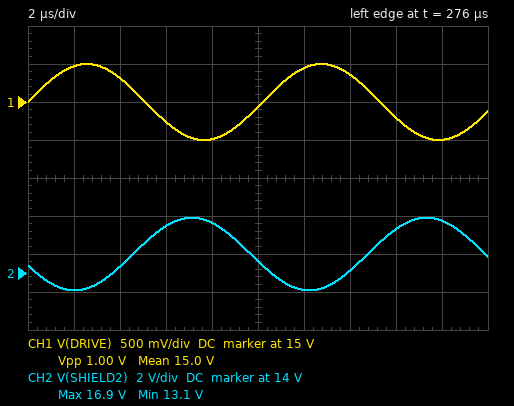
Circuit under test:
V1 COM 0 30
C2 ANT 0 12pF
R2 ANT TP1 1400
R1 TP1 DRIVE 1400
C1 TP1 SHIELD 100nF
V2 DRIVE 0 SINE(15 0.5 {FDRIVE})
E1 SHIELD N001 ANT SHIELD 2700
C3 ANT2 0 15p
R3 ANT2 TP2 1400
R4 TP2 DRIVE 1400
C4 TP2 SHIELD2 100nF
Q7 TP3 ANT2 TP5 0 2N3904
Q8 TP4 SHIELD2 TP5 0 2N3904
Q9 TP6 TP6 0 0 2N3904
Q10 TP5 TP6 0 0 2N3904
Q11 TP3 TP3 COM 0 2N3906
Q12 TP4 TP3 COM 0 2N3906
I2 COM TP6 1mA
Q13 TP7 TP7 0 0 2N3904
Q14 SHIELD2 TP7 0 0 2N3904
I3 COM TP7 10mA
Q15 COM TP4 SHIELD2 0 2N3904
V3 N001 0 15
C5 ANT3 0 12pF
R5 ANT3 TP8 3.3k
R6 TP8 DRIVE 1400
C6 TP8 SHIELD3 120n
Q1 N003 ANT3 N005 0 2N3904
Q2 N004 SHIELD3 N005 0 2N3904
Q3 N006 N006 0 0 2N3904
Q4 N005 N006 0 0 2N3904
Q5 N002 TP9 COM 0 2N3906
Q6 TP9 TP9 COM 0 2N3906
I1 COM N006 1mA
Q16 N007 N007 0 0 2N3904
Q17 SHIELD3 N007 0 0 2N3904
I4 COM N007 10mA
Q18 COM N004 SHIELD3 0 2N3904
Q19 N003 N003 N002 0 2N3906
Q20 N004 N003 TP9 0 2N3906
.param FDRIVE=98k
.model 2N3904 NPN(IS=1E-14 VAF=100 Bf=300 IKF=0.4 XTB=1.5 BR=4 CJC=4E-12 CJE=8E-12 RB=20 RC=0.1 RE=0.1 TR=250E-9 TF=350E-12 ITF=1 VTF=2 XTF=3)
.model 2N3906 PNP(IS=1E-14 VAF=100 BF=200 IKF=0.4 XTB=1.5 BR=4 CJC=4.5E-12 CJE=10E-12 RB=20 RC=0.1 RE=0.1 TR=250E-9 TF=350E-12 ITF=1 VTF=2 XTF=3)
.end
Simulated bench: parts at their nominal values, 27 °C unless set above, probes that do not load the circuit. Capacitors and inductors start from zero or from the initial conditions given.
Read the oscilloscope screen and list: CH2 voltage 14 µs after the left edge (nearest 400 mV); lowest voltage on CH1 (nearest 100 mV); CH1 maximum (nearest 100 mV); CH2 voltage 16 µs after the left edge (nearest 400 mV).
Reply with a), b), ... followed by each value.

a) 14.0 V
b) 14.5 V
c) 15.5 V
d) 16.4 V
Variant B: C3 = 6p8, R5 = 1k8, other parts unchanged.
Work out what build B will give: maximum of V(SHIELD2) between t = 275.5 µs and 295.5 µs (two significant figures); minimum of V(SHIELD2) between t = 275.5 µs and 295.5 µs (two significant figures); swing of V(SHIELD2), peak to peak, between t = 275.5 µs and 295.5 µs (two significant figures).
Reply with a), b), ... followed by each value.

a) 16 V
b) 14 V
c) 2.7 V
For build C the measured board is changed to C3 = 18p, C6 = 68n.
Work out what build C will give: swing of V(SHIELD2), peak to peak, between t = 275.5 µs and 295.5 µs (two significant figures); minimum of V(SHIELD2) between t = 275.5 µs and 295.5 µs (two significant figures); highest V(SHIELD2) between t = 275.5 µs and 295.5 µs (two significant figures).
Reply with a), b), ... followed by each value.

a) 2.1 V
b) 14 V
c) 16 V
